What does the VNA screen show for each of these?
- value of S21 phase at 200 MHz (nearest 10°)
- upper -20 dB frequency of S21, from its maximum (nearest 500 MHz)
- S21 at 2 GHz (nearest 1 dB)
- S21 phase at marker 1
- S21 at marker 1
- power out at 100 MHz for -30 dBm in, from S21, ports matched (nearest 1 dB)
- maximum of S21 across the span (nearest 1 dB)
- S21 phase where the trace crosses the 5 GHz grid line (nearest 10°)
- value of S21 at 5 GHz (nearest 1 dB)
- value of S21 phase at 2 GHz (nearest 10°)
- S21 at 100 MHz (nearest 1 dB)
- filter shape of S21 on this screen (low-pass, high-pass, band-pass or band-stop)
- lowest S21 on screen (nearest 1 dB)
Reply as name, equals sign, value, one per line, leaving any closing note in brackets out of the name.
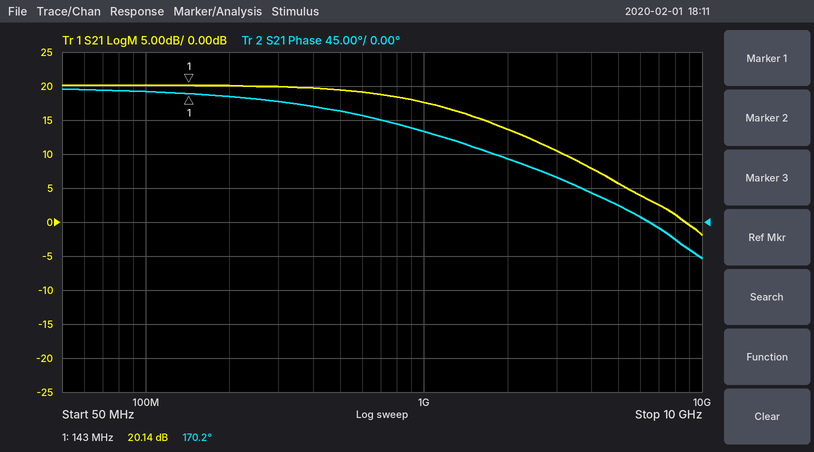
value of S21 phase at 200 MHz = 170°
upper -20 dB frequency of S21, from its maximum = 8.5 GHz
S21 at 2 GHz = 14 dB
S21 phase at marker 1 = 170.2°
S21 at marker 1 = 20.14 dB
power out at 100 MHz for -30 dBm in, from S21, ports matched = -10 dBm
maximum of S21 across the span = 20 dB
S21 phase where the trace crosses the 5 GHz grid line = 20°
value of S21 at 5 GHz = 6 dB
value of S21 phase at 2 GHz = 80°
S21 at 100 MHz = 20 dB
filter shape of S21 on this screen = low-pass
lowest S21 on screen = -2 dB
